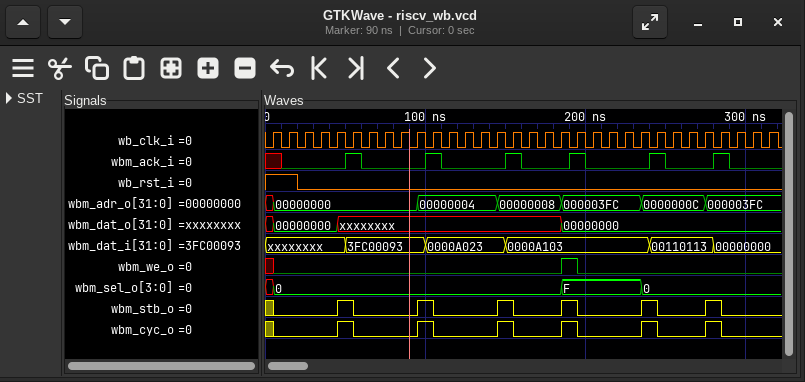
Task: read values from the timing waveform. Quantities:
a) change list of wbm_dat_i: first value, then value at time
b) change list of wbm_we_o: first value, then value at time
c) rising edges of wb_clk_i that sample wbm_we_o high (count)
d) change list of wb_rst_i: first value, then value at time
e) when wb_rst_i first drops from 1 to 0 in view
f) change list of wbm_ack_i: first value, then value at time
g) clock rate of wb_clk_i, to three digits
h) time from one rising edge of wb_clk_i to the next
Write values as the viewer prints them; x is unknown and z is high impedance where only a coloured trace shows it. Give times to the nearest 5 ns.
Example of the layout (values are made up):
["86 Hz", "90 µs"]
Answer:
["xxxxxxxx, 3FC00093 at 50 ns, 0000A023 at 100 ns, 0000A103 at 150 ns, 00110113 at 240 ns, 00000000 at 280 ns", "x, 0 at 5 ns, 1 at 185 ns, 0 at 195 ns", "1", "1, 0 at 20 ns", "20 ns", "x, 0 at 10 ns, 1 at 50 ns, 0 at 60 ns, 1 at 100 ns, 0 at 110 ns, 1 at 150 ns, 0 at 160 ns, 1 at 190 ns, 0 at 200 ns, 1 at 240 ns, 0 at 250 ns, 1 at 280 ns, 0 at 290 ns", "100 MHz", "10 ns"]
